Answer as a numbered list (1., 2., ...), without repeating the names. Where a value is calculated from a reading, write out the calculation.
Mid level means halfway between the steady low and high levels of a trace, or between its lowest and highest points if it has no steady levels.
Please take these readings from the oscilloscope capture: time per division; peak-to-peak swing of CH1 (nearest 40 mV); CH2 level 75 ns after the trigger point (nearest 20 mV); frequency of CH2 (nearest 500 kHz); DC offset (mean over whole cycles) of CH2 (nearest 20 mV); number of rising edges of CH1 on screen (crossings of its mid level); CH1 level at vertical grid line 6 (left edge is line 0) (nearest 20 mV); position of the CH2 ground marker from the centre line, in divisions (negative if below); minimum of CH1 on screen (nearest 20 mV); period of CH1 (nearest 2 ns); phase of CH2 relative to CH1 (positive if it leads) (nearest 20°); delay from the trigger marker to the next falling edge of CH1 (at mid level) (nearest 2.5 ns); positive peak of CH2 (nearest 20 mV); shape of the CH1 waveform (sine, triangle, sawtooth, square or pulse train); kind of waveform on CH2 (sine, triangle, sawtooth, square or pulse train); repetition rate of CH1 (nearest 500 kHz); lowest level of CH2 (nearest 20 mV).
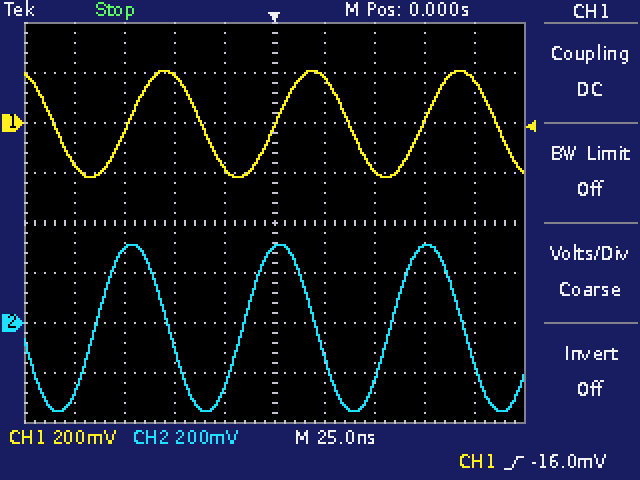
1. 25 ns
2. 440 mV
3. 300 mV
4. 13.5 MHz
5. (320 mV + (-360 mV)) / 2 ≈ -20 mV
6. 3
7. 180 mV
8. -2.0 div
9. -220 mV
10. 74 ns
11. +80°
12. 37.5 ns
13. 320 mV
14. sine
15. sine
16. 1 / 74 ns ≈ 13.5 MHz
17. -360 mV
